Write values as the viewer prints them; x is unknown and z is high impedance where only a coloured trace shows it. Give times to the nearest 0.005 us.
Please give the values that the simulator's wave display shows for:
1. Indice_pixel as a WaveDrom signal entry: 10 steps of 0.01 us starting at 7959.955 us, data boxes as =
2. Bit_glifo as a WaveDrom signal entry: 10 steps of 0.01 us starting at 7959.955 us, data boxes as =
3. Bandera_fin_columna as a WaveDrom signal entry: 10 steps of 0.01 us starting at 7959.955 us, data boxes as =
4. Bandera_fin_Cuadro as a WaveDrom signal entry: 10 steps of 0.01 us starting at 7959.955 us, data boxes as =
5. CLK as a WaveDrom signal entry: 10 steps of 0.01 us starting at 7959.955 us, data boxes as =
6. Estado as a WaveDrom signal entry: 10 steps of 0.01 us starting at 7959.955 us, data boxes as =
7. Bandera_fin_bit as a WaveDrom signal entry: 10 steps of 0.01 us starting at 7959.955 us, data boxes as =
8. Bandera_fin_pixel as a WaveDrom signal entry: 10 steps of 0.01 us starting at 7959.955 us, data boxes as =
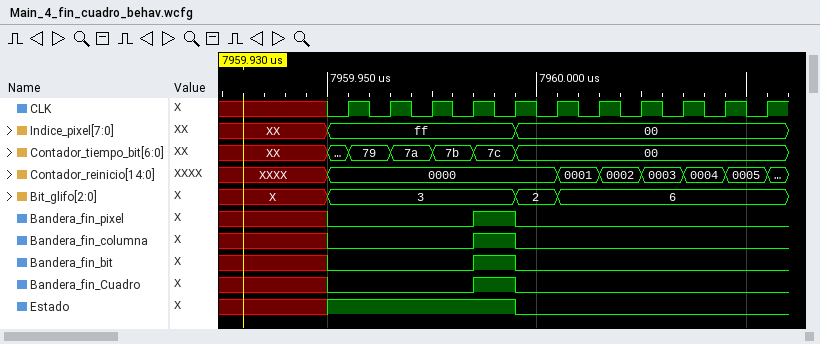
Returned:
{name: 'Indice_pixel', wave: '=...=.....', data: 'ff 00'}
{name: 'Bit_glifo', wave: '=...==....', data: '3 2 6'}
{name: 'Bandera_fin_columna', wave: '0..10.....'}
{name: 'Bandera_fin_Cuadro', wave: '0..10.....'}
{name: 'CLK', wave: 'p.........'}
{name: 'Estado', wave: '1...0.....'}
{name: 'Bandera_fin_bit', wave: '0..10.....'}
{name: 'Bandera_fin_pixel', wave: '0..10.....'}
